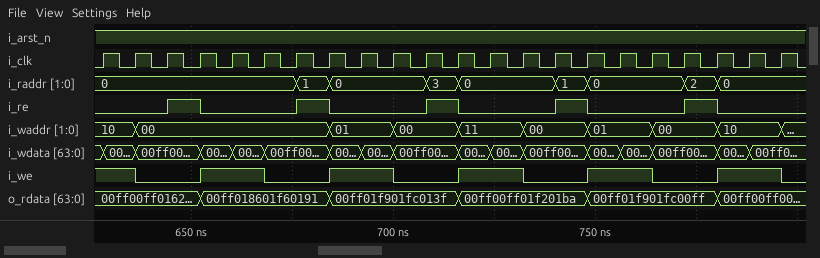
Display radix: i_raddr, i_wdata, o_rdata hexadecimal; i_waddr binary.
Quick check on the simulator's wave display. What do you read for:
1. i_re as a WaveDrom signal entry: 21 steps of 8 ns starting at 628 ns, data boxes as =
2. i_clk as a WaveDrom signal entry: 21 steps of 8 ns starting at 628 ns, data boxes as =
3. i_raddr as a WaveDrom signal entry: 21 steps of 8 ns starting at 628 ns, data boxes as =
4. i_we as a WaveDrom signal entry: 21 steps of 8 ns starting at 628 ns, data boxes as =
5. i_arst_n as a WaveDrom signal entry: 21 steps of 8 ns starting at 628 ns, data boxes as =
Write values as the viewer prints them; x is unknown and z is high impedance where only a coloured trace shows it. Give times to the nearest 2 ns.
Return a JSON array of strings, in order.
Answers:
["{name: 'i_re', wave: '0.10..10..10..10..10.'}", "{name: 'i_clk', wave: 'p....................'}", "{name: 'i_raddr', wave: '=.....==..==..==..==.', data: '0 1 0 3 0 1 0 2 0'}", "{name: 'i_we', wave: '10.1.0.1.0.1.0.1.0.1.'}", "{name: 'i_arst_n', wave: '1....................'}"]
